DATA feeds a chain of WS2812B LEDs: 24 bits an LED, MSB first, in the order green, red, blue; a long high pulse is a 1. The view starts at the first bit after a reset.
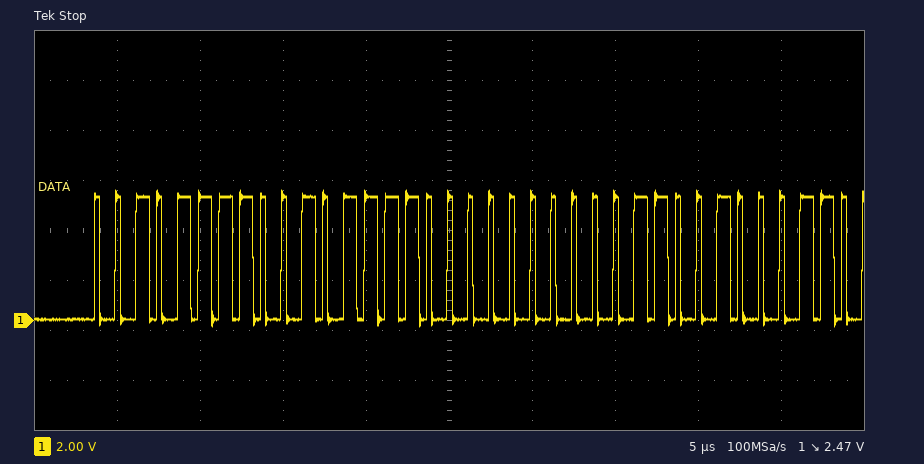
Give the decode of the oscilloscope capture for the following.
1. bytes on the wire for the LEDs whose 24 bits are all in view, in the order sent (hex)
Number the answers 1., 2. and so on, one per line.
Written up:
1. 2F 2F 00
